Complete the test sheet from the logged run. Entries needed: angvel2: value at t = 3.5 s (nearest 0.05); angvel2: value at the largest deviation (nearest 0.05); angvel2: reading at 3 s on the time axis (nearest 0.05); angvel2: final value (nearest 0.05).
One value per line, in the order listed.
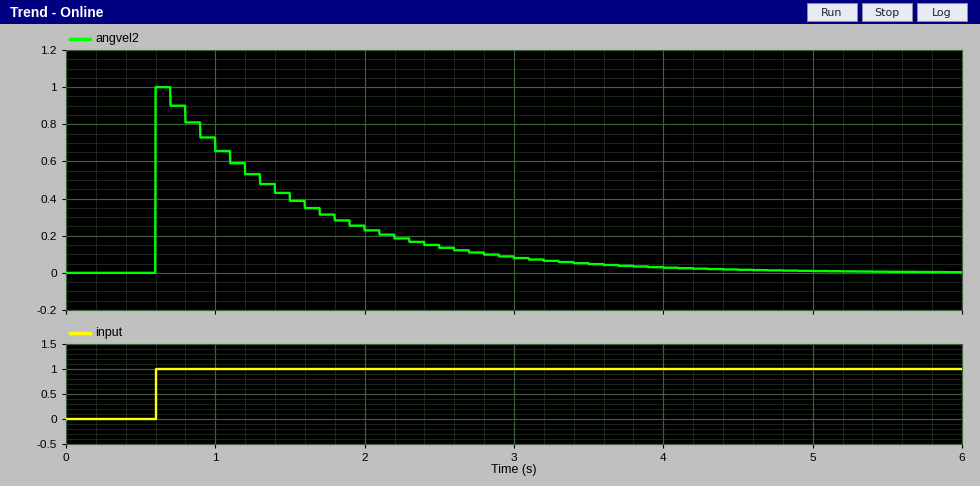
0.05
1.00
0.10
0.00
